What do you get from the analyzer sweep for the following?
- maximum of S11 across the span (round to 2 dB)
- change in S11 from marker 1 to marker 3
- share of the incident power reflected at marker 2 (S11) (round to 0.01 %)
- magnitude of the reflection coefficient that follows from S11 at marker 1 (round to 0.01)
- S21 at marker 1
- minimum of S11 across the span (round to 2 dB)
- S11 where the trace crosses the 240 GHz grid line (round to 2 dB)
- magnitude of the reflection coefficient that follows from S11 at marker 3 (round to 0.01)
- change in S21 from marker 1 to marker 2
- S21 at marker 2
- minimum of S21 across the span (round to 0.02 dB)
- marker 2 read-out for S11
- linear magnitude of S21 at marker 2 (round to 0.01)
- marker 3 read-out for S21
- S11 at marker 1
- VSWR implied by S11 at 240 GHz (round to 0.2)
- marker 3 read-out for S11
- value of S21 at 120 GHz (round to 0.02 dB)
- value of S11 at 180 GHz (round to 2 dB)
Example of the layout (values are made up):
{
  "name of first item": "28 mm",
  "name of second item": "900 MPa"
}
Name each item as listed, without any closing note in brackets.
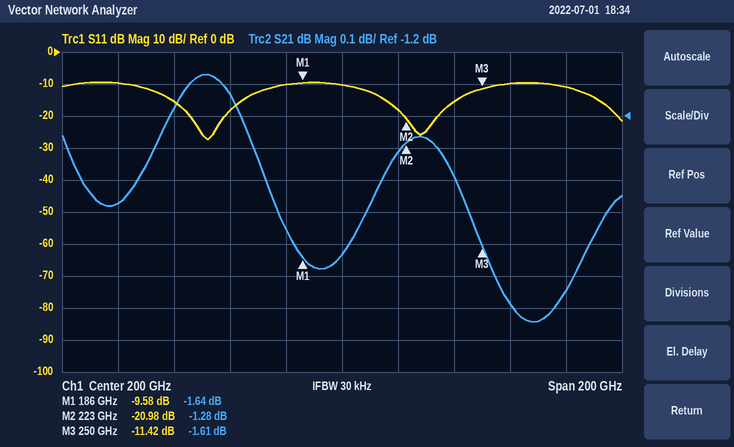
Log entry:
{
  "maximum of S11 across the span": "-10 dB",
  "change in S11 from marker 1 to marker 3": "-1.84 dB",
  "share of the incident power reflected at marker 2 (S11)": "0.80 %",
  "magnitude of the reflection coefficient that follows from S11 at marker 1": "0.33",
  "S21 at marker 1": "-1.64 dB",
  "minimum of S11 across the span": "-28 dB",
  "S11 where the trace crosses the 240 GHz grid line": "-16 dB",
  "magnitude of the reflection coefficient that follows from S11 at marker 3": "0.27",
  "change in S21 from marker 1 to marker 2": "0.36 dB",
  "S21 at marker 2": "-1.28 dB",
  "minimum of S21 across the span": "-1.84 dB",
  "marker 2 read-out for S11": "-20.98 dB",
  "linear magnitude of S21 at marker 2": "0.86",
  "marker 3 read-out for S21": "-1.61 dB",
  "S11 at marker 1": "-9.58 dB",
  "VSWR implied by S11 at 240 GHz": "1.4",
  "marker 3 read-out for S11": "-11.42 dB",
  "value of S21 at 120 GHz": "-1.48 dB",
  "value of S11 at 180 GHz": "-10 dB"
}
